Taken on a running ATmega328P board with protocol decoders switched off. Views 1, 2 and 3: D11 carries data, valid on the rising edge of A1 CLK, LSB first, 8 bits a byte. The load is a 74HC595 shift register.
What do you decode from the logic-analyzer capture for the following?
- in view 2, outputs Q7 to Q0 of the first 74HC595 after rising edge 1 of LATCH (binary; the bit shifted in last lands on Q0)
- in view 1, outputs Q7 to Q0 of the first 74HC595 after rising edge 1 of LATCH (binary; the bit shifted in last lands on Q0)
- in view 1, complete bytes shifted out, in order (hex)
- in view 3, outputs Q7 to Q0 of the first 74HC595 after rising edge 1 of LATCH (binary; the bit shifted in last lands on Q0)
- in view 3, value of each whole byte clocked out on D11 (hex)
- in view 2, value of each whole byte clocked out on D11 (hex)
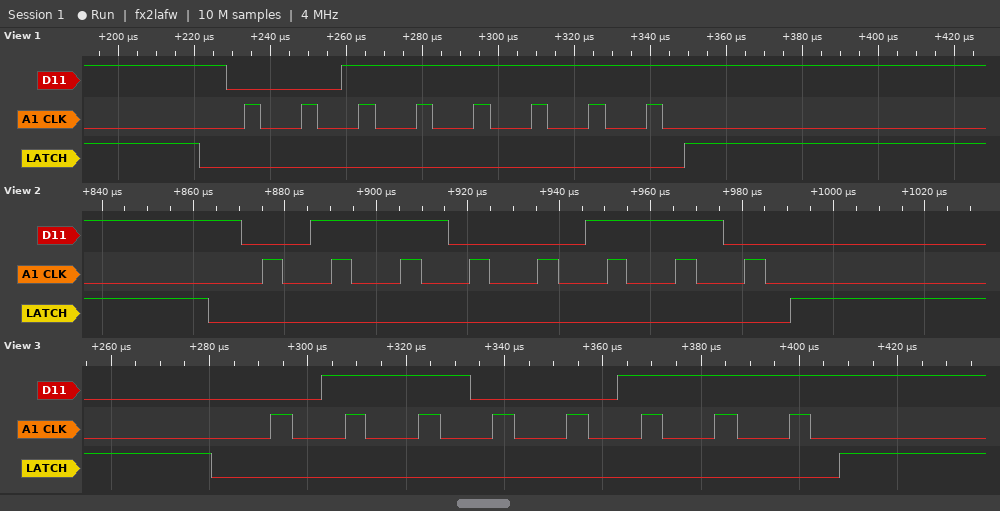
01100110
00111111
FC
01100111
E6
66
